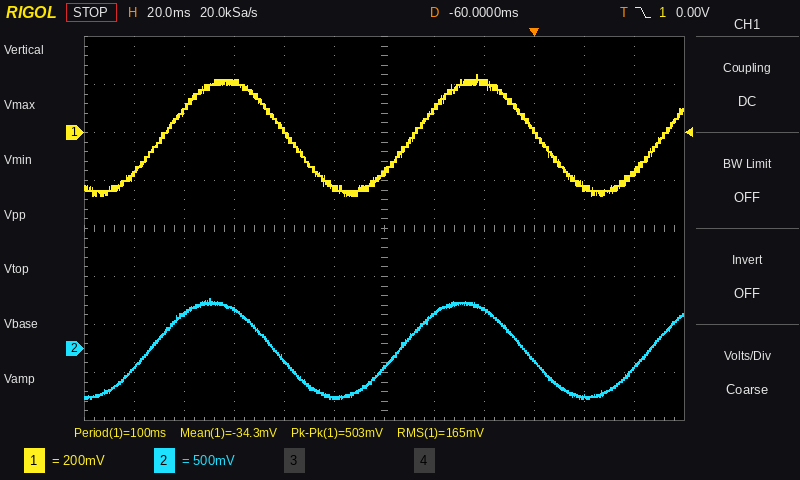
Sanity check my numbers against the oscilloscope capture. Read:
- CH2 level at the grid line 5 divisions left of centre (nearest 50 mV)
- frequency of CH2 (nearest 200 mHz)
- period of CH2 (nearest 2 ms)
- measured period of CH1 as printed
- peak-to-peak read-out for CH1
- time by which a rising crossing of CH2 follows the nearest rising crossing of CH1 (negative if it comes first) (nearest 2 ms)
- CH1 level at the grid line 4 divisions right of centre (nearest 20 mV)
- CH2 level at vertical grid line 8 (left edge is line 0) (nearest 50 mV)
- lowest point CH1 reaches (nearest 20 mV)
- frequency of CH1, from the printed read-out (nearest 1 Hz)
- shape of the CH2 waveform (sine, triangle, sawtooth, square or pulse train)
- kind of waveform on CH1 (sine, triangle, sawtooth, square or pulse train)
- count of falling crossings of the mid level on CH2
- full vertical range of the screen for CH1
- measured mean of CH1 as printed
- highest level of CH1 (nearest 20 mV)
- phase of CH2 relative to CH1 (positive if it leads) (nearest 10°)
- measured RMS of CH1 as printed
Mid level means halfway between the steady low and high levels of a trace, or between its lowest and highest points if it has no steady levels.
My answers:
-200 mV
10.0 Hz
100 ms
100 ms
503 mV
-6 ms
-220 mV
400 mV
-260 mV
10 Hz
sine
sine
2
1.6 V
-34.3 mV
240 mV
+20°
165 mV
